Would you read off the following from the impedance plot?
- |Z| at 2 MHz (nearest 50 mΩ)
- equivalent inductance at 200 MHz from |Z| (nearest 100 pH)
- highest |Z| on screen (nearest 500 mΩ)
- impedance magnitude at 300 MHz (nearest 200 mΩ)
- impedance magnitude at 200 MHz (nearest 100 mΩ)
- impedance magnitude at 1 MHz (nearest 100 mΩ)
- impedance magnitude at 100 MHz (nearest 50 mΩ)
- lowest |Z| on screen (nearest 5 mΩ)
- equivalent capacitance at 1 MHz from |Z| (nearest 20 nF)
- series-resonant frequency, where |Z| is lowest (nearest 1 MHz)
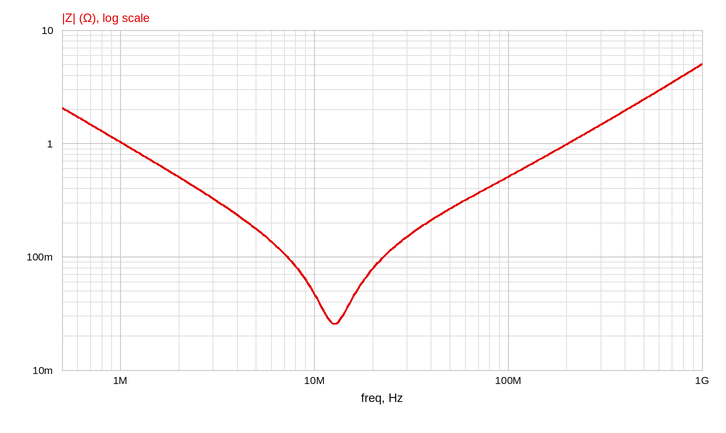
500 mΩ
800 pH
5.0 Ω
1.4 Ω
1.0 Ω
1.0 Ω
500 mΩ
25 mΩ
160 nF
13 MHz
